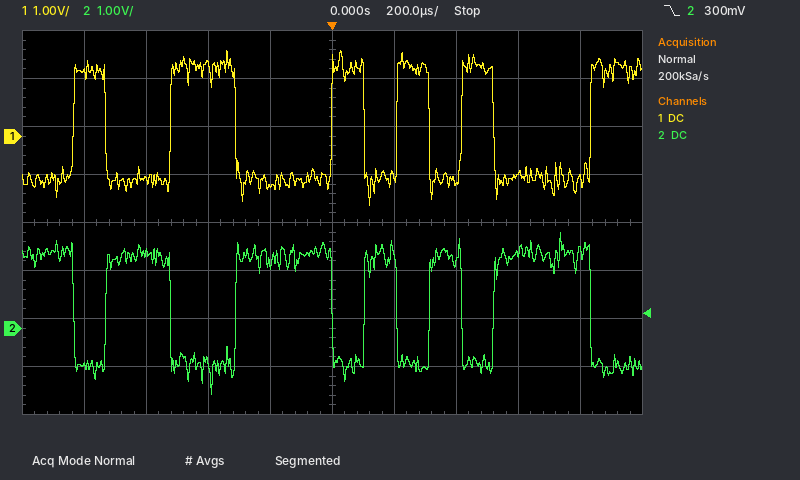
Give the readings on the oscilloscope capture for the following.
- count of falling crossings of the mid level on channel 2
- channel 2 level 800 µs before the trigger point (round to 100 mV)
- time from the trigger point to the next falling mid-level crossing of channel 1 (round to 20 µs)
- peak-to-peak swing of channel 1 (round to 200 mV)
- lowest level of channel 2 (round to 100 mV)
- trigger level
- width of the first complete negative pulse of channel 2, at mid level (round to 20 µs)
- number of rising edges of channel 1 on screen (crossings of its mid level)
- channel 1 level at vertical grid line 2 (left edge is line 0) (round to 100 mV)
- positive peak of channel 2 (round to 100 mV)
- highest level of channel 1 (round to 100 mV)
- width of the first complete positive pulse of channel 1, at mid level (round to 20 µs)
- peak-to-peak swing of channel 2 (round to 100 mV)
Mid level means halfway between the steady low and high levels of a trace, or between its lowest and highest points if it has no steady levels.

6
-800 mV
100 µs
3.2 V
-1.4 V
300 mV
100 µs
6
-900 mV
2.0 V
1.8 V
100 µs
3.4 V
